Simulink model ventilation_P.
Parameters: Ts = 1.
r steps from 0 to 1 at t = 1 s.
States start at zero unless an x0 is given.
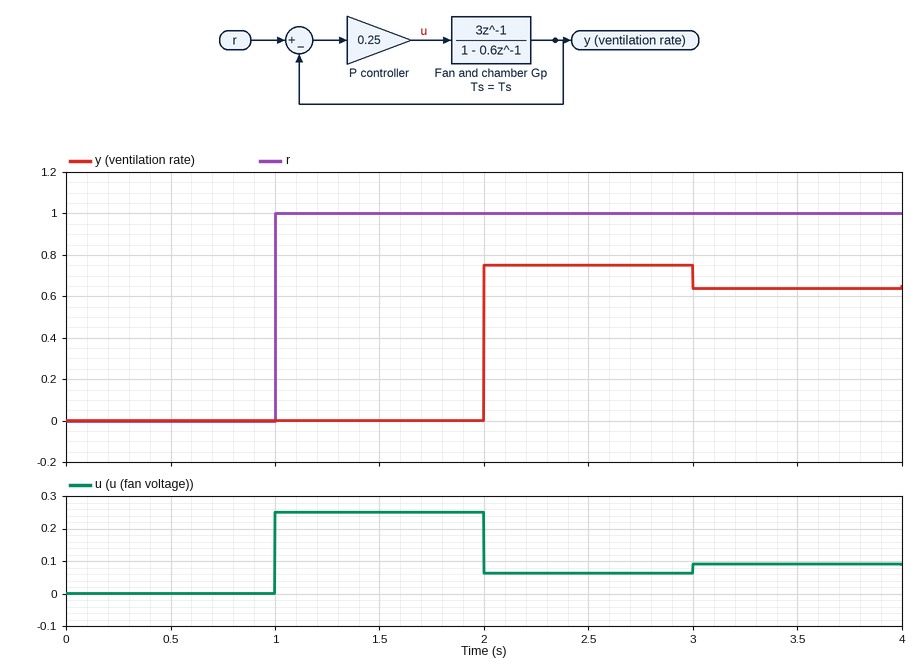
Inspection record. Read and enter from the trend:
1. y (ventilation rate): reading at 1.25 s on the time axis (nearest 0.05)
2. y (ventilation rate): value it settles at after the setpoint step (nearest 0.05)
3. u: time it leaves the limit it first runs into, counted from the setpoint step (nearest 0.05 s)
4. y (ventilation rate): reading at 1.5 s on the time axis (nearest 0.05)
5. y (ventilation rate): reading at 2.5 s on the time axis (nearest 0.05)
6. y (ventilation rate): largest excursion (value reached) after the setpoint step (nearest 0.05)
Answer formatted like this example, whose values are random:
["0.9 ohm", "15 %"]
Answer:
["0.00", "0.65", "1.00 s", "0.00", "0.75", "0.75"]
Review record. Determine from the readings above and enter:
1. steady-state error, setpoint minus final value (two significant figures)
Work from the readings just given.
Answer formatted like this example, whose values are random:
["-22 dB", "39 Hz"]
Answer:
["0.35"]
